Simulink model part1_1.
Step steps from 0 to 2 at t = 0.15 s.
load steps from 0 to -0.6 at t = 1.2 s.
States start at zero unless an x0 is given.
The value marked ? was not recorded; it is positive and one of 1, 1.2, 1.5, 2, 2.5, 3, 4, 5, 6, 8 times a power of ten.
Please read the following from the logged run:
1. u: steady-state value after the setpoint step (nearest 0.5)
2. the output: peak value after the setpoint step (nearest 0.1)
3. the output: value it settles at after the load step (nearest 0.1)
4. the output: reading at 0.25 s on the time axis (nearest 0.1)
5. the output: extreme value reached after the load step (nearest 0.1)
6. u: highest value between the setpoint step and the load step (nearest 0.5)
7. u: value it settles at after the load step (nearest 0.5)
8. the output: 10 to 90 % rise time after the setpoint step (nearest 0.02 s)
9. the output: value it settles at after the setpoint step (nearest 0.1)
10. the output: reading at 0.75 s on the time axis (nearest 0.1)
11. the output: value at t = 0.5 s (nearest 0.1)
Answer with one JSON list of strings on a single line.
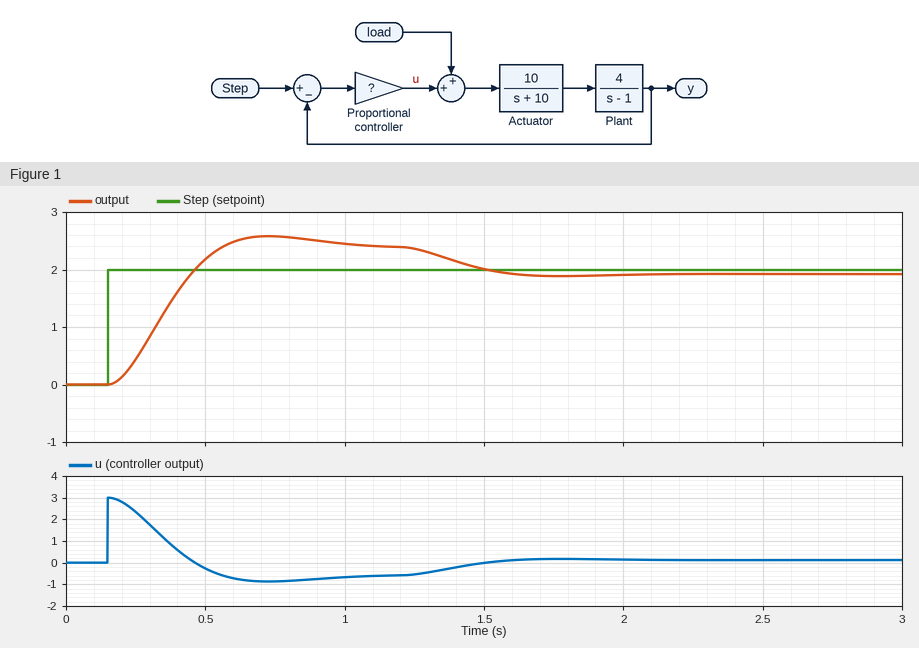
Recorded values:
["-0.5", "2.6", "1.9", "0.4", "1.9", "3.0", "0.0", "0.28 s", "2.4", "2.6", "2.2"]
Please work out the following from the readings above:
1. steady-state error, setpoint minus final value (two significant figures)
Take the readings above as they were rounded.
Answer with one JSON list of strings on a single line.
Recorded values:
["-0.40"]
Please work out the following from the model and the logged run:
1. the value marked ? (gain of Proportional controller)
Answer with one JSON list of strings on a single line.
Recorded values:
["1.5"]
